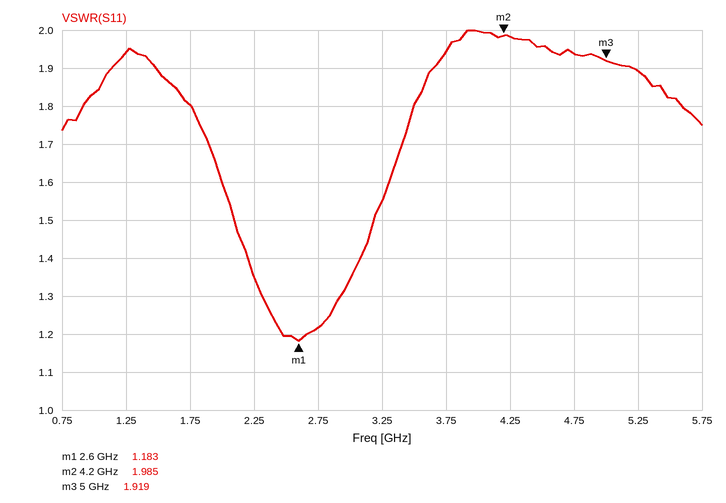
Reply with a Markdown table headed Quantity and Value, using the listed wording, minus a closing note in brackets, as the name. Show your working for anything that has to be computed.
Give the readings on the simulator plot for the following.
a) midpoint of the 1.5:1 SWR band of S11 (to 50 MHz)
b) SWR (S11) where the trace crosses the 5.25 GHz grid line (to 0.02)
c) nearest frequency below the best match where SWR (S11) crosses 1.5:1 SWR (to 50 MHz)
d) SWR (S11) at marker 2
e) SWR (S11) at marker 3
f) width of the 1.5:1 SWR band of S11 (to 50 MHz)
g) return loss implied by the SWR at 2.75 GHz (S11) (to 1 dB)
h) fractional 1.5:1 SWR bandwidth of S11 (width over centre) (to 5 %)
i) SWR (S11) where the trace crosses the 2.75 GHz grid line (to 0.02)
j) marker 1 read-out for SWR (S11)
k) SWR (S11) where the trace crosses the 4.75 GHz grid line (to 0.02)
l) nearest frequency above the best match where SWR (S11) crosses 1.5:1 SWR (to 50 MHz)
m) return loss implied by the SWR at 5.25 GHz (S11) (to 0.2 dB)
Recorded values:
| Quantity | Value |
|---|---|
| midpoint of the 1.5:1 SWR band of S11 | 2.65 GHz |
| SWR (S11) where the trace crosses the 5.25 GHz grid line | 1.90 |
| nearest frequency below the best match where SWR (S11) crosses 1.5:1 SWR | 2.10 GHz |
| SWR (S11) at marker 2 | 1.985 |
| SWR (S11) at marker 3 | 1.919 |
| width of the 1.5:1 SWR band of S11 | 3.20 GHz − 2.10 GHz = 1.10 GHz |
| return loss implied by the SWR at 2.75 GHz (S11) | −20 log10((1.22 − 1)/(1.22 + 1)) ≈ 20 dB |
| fractional 1.5:1 SWR bandwidth of S11 (width over centre) | 1.1 GHz / 2.65 GHz ≈ 41.5 %, so 40 % to the nearest 5 % |
| SWR (S11) where the trace crosses the 2.75 GHz grid line | 1.22 |
| marker 1 read-out for SWR | 1.183 |
| SWR (S11) where the trace crosses the 4.75 GHz grid line | 1.94 |
| nearest frequency above the best match where SWR (S11) crosses 1.5:1 SWR | 3.20 GHz |
| return loss implied by the SWR at 5.25 GHz (S11) | −20 log10((1.9 − 1)/(1.9 + 1)) ≈ 10.2 dB |
